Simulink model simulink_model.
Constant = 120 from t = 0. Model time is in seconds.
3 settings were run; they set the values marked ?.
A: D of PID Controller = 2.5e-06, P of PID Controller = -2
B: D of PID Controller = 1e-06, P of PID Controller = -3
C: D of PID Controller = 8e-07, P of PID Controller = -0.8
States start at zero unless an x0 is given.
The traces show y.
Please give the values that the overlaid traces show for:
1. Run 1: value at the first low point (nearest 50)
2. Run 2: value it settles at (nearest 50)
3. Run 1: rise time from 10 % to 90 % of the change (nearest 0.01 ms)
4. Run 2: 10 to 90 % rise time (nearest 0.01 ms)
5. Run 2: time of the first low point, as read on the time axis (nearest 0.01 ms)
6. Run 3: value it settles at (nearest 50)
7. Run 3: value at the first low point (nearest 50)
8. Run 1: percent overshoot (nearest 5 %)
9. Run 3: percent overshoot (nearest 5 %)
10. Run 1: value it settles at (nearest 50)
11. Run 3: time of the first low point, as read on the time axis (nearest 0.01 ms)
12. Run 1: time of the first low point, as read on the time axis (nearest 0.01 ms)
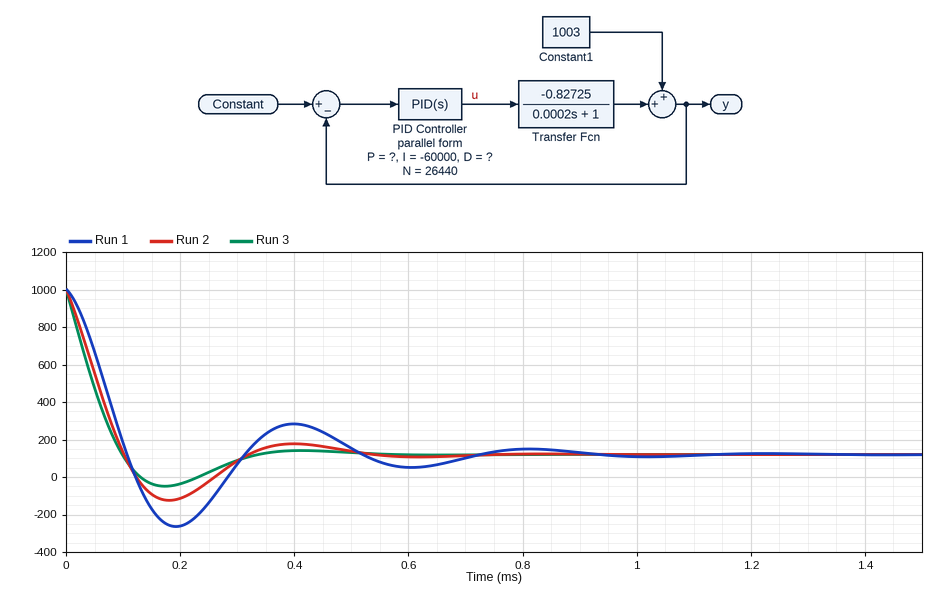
-250
100
0.08 ms
0.08 ms
0.18 ms
100
-50
45 %
20 %
100
0.17 ms
0.19 ms
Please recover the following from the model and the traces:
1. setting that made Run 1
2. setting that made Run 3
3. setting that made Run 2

C
B
A
